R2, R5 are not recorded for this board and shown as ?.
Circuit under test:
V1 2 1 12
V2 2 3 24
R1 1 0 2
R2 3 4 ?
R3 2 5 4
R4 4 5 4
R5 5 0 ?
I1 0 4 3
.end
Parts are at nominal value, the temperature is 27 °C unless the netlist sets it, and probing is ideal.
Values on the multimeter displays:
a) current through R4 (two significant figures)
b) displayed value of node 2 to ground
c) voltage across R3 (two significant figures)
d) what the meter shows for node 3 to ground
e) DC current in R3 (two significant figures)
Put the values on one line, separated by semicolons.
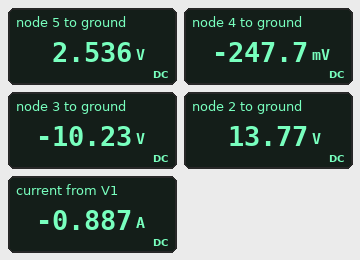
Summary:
700 mA; 13.77 V; 11 V; -10.23 V; 2.8 A
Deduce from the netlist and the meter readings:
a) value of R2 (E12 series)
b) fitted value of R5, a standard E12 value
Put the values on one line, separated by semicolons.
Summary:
2.7 Ω; 1.2 Ω
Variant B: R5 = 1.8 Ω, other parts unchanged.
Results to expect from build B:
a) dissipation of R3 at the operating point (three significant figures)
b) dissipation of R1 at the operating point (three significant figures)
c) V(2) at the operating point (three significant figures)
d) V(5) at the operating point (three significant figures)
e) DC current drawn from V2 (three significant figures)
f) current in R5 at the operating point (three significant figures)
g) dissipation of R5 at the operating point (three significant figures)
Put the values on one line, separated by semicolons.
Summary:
28.8 W; 2.37 W; 14.2 V; 3.44 V; 3.77 A; 1.91 A; 6.58 W
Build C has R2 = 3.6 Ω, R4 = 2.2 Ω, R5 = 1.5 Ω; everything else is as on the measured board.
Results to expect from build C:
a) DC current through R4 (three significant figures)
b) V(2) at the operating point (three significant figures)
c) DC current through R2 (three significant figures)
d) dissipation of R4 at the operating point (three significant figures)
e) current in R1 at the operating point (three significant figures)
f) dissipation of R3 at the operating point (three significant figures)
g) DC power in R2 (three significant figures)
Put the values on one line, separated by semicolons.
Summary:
470 mA; 13.7 V; 3.47 A; 485 mW; 850 mA; 27.4 W; 43.3 W
